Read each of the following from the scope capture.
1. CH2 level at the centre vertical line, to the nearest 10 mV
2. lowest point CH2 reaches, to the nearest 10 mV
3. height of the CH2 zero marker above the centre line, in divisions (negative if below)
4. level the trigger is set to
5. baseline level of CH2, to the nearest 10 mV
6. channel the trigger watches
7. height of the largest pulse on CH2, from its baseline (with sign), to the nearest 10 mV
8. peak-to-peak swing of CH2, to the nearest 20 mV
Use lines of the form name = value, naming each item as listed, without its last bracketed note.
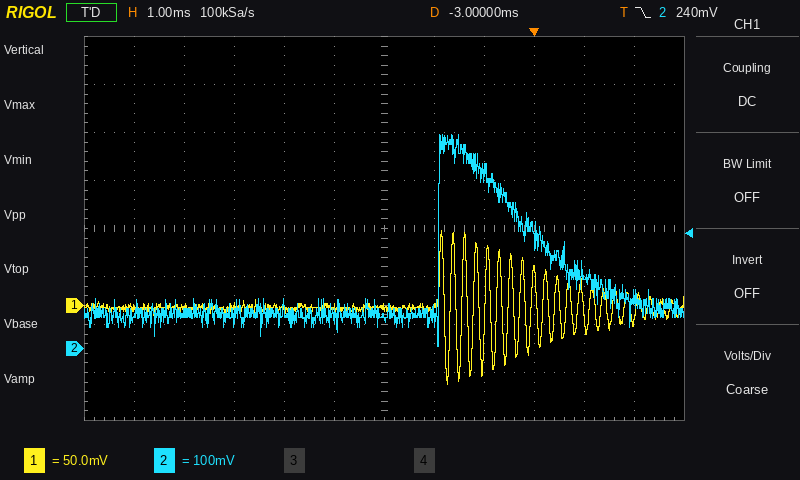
CH2 level at the centre vertical line, to the nearest 10 mV = 60 mV
lowest point CH2 reaches, to the nearest 10 mV = 0 mV
height of the CH2 zero marker above the centre line, in divisions = -2.5 div
level the trigger is set to = 240 mV
baseline level of CH2, to the nearest 10 mV = 70 mV
channel the trigger watches = CH2
height of the largest pulse on CH2, from its baseline (with sign), to the nearest 10 mV = +370 mV
peak-to-peak swing of CH2, to the nearest 20 mV = 440 mV
